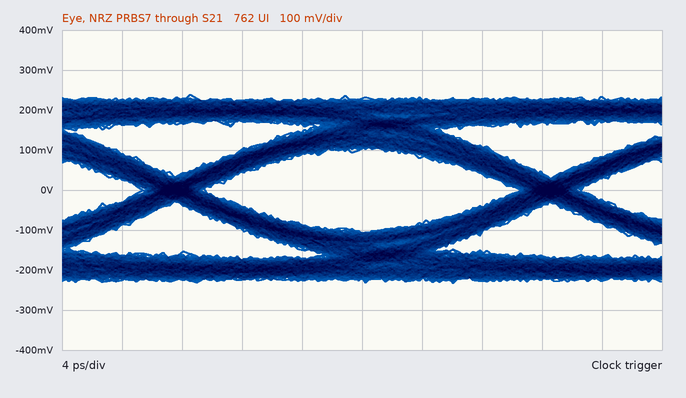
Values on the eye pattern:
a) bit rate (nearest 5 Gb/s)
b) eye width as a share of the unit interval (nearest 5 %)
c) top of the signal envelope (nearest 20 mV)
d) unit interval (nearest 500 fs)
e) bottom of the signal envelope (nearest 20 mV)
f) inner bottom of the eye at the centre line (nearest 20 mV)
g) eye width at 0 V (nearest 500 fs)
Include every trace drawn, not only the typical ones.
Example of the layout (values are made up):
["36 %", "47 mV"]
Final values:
["40 Gb/s", "85 %", "240 mV", "25.0 ps", "-240 mV", "-100 mV", "21.0 ps"]
